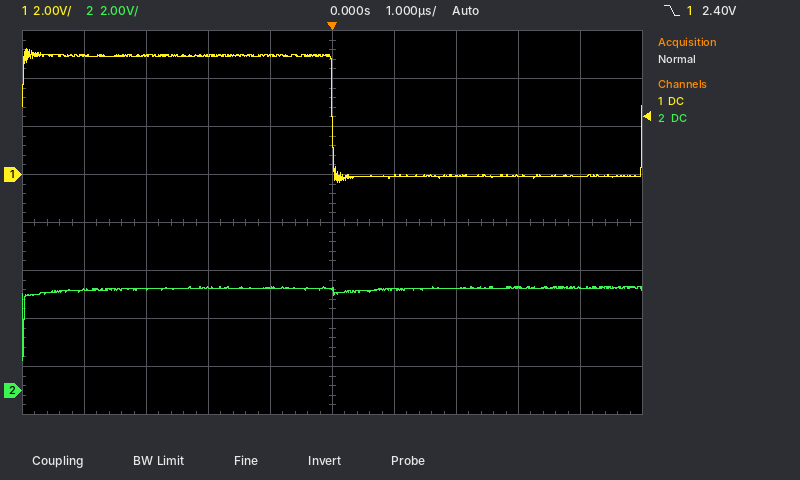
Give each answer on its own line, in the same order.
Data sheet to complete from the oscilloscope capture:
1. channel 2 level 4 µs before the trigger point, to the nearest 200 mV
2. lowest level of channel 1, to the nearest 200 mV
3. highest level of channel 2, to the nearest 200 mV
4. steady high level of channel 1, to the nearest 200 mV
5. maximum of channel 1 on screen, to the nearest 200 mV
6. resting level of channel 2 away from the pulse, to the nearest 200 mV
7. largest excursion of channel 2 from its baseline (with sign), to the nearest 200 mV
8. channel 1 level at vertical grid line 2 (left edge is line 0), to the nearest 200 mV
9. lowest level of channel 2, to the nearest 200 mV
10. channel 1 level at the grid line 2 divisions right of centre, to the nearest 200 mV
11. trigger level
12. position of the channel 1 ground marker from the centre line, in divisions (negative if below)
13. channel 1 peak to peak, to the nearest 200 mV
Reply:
4.2 V
-400 mV
4.4 V
5.0 V
5.2 V
4.2 V
-3.0 V
5.0 V
1.2 V
0.0 V
2.40 V
+1.0 div
5.6 V
